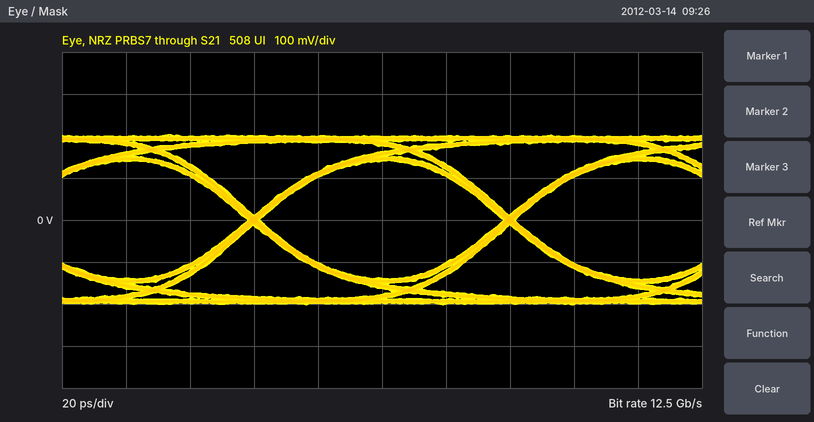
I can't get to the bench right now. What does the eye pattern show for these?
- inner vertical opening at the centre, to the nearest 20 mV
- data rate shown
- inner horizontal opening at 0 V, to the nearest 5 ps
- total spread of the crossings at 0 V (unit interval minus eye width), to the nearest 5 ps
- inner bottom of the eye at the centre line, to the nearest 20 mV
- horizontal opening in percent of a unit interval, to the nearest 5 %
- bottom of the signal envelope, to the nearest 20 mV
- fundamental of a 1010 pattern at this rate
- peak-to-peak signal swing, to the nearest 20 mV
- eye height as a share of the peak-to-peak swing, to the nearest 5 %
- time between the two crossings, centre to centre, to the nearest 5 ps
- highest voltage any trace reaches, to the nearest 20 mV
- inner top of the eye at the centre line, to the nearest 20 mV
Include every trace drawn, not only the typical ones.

280 mV
12.5 Gb/s
75 ps
5 ps
-140 mV
95 %
-200 mV
6.25 GHz
400 mV
70 %
80 ps
200 mV
140 mV
